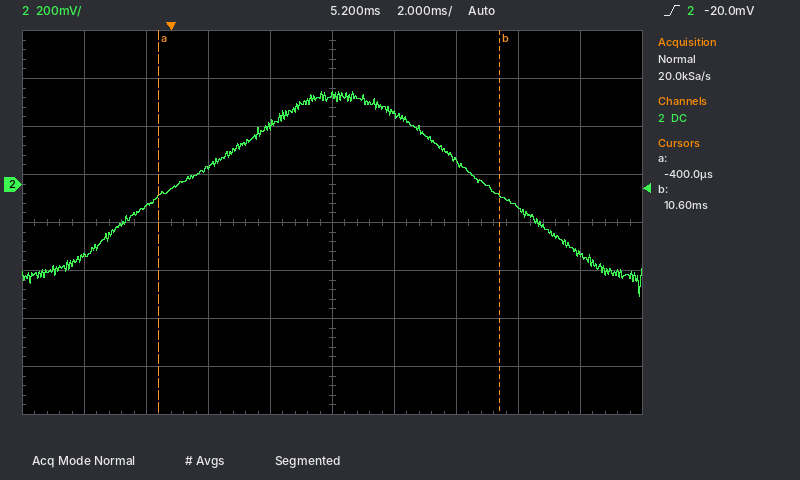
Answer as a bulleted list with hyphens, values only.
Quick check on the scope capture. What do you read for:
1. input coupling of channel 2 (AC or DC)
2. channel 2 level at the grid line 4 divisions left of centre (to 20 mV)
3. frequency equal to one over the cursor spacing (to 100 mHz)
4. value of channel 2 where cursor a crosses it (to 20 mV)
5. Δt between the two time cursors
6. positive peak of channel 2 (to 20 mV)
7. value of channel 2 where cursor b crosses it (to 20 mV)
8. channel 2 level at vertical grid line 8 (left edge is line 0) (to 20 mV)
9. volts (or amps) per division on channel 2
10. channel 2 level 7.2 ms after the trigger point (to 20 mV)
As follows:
- DC
- -300 mV
- 90.9 Hz
- -40 mV
- 11.0 ms
- 380 mV
- -40 mV
- -100 mV
- 200 mV
- 300 mV
